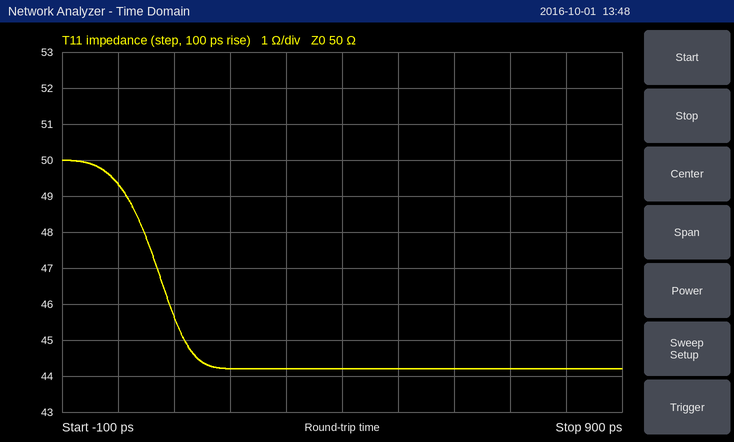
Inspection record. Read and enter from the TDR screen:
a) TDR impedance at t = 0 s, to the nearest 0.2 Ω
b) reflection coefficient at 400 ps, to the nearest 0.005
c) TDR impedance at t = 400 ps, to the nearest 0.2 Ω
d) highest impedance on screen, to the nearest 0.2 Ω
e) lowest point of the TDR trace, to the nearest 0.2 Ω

49.4 Ω
-0.060
44.2 Ω
50.0 Ω
44.2 Ω
